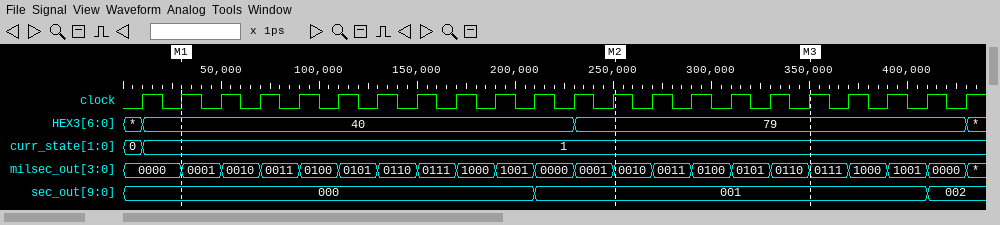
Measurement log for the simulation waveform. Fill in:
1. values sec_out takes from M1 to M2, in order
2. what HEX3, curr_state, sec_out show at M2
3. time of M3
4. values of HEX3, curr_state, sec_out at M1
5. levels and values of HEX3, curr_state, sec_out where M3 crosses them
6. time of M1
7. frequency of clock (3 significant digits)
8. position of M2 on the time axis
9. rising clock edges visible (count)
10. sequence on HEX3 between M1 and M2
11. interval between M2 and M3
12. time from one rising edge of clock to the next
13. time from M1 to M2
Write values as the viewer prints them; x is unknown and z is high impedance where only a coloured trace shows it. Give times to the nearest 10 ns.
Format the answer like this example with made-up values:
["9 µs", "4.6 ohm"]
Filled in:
["000, 001", "HEX3=79, curr_state=1, sec_out=001", "350 ns", "HEX3=40, curr_state=1, sec_out=000", "HEX3=79, curr_state=1, sec_out=001", "30 ns", "50.0 MHz", "250 ns", "22", "40, 79", "100 ns", "20 ns", "220 ns"]
